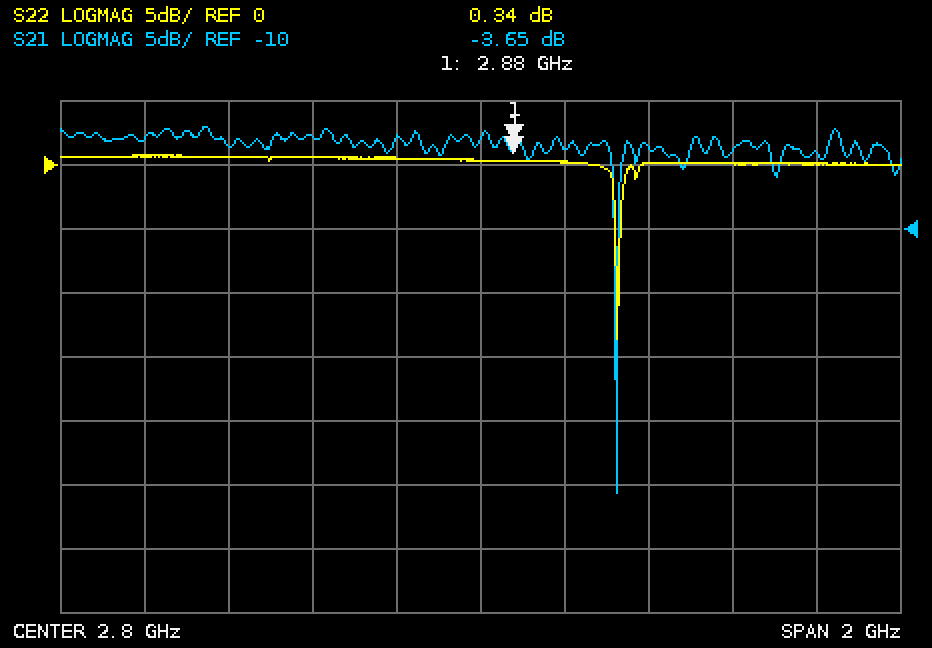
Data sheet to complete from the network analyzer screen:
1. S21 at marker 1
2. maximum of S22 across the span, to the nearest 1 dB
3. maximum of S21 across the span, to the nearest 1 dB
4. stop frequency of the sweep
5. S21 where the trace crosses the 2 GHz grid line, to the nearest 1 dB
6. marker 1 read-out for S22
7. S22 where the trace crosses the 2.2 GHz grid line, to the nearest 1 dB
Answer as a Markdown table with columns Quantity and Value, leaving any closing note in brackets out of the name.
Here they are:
| Quantity | Value |
|---|---|
| S21 at marker 1 | -3.65 dB |
| maximum of S22 across the span, to the nearest 1 dB | 1 dB |
| maximum of S21 across the span, to the nearest 1 dB | -2 dB |
| stop frequency of the sweep | 3.8 GHz |
| S21 where the trace crosses the 2 GHz grid line, to the nearest 1 dB | -3 dB |
| marker 1 read-out for S22 | 0.34 dB |
| S22 where the trace crosses the 2.2 GHz grid line, to the nearest 1 dB | 1 dB |
